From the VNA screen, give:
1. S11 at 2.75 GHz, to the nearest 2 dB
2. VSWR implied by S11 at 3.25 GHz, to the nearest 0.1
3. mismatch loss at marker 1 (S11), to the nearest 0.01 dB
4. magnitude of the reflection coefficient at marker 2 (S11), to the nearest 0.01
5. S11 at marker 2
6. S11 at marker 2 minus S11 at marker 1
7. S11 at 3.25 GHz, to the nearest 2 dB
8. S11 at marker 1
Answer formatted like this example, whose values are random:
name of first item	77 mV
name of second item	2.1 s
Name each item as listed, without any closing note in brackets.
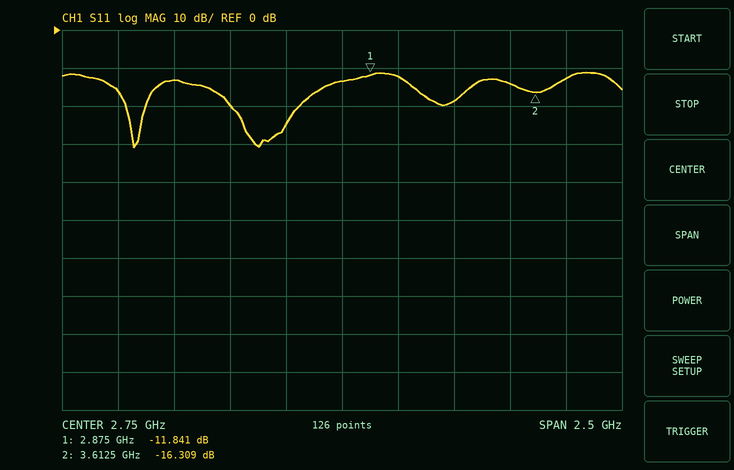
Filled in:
S11 at 2.75 GHz, to the nearest 2 dB	-14 dB
VSWR implied by S11 at 3.25 GHz, to the nearest 0.1	1.3
mismatch loss at marker 1 (S11), to the nearest 0.01 dB	0.29 dB
magnitude of the reflection coefficient at marker 2 (S11), to the nearest 0.01	0.15
S11 at marker 2	-16.309 dB
S11 at marker 2 minus S11 at marker 1	-4.468 dB
S11 at 3.25 GHz, to the nearest 2 dB	-18 dB
S11 at marker 1	-11.841 dB
